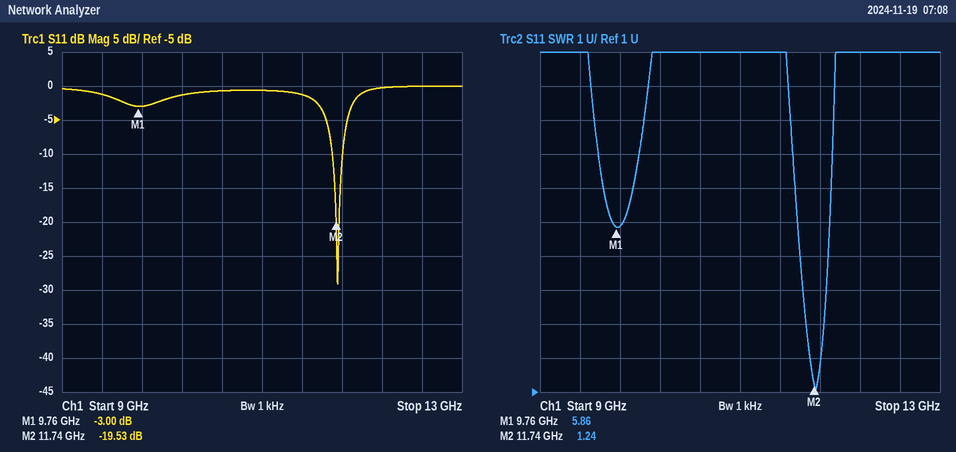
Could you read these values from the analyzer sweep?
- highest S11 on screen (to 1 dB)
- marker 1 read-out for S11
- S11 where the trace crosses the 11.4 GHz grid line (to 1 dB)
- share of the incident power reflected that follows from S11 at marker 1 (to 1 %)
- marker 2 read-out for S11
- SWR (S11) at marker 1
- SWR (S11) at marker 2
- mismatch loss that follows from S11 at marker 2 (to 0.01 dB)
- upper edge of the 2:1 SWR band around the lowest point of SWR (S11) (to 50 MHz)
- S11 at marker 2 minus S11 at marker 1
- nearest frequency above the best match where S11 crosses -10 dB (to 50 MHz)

0 dB
-3.00 dB
-1 dB
50 %
-19.53 dB
5.86
1.24
0.05 dB
11.80 GHz
-16.53 dB
11.80 GHz
